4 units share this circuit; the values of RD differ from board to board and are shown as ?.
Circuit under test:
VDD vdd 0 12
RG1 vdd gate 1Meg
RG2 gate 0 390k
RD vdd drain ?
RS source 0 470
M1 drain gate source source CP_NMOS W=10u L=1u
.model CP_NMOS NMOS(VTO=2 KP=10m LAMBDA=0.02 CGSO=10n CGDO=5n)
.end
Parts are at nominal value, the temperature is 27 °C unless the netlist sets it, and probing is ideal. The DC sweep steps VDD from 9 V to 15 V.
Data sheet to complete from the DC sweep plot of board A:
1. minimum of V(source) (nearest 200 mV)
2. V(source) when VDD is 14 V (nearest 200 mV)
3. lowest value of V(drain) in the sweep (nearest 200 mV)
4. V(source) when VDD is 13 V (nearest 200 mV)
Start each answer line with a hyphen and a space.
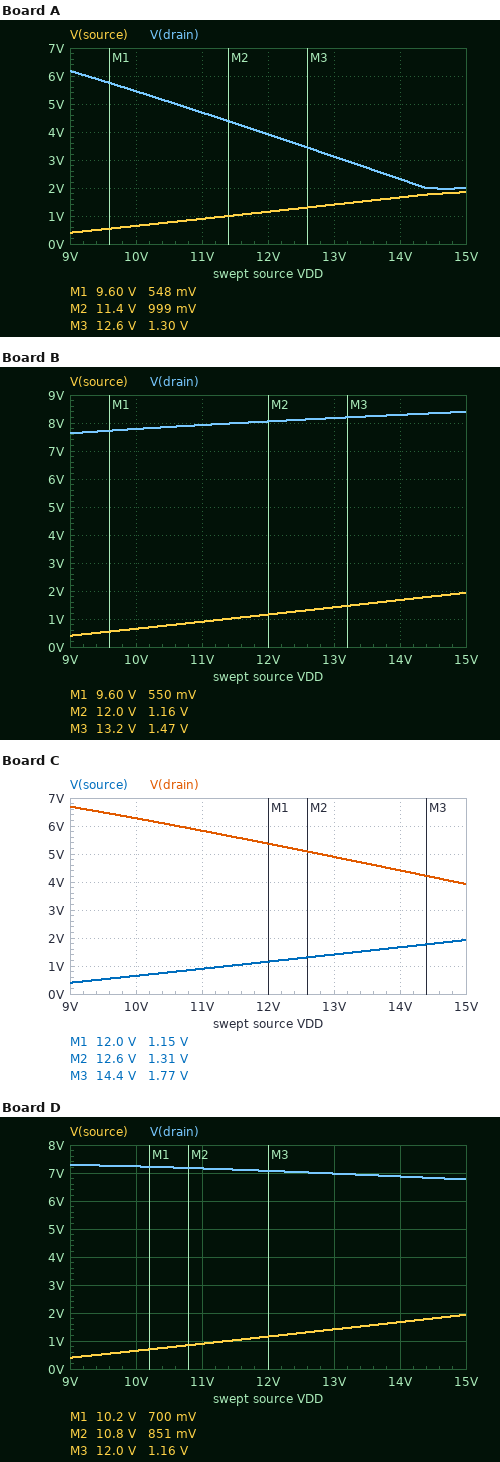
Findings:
- 400 mV
- 1.6 V
- 2.0 V
- 1.4 V
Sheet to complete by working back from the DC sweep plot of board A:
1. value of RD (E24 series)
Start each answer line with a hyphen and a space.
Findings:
- 3.3 kΩ
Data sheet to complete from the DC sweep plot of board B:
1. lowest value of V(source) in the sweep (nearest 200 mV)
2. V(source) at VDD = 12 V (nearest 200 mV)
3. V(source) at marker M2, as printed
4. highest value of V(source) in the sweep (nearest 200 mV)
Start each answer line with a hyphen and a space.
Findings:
- 400 mV
- 1.2 V
- 1.16 V
- 2.0 V
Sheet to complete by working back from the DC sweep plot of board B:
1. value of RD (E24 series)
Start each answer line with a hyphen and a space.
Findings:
- 1.6 kΩ
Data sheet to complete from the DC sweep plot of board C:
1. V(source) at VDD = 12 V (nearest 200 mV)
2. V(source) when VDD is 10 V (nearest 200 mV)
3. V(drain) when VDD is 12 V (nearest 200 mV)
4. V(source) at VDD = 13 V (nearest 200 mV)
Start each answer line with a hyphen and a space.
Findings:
- 1.2 V
- 600 mV
- 5.4 V
- 1.4 V
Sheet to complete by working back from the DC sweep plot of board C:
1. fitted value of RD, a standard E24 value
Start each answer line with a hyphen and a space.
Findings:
- 2.7 kΩ
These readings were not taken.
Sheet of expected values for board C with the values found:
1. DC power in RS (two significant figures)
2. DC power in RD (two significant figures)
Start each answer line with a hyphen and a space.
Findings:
- 2.8 mW
- 16 mW
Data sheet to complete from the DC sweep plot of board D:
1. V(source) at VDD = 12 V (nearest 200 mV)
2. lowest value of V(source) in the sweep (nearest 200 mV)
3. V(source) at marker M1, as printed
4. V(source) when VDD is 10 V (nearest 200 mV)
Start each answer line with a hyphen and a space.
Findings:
- 1.2 V
- 400 mV
- 700 mV
- 600 mV
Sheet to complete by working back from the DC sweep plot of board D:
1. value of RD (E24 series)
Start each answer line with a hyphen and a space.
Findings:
- 2 kΩ
